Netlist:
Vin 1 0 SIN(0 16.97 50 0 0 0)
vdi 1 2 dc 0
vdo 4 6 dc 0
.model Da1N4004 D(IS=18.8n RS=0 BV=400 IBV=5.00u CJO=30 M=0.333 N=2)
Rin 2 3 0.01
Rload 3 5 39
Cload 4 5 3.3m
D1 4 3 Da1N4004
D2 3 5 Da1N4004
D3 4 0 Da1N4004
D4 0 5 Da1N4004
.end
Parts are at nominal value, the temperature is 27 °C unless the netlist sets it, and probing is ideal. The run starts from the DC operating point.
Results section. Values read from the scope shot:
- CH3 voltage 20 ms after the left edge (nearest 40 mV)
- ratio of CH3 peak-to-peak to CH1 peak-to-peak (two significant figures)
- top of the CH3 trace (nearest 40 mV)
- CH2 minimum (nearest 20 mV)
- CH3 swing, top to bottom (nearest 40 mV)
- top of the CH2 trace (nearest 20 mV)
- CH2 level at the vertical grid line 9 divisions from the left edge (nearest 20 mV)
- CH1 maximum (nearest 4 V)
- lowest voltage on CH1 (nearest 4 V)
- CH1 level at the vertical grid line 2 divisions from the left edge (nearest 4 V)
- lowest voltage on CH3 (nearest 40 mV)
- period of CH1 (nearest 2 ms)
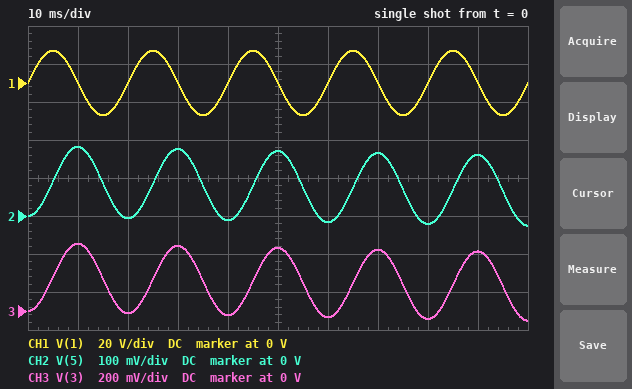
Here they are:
0 V
0.012
360 mV
-20 mV
400 mV
180 mV
160 mV
16 V
-16 V
0 V
-40 mV
20 ms
